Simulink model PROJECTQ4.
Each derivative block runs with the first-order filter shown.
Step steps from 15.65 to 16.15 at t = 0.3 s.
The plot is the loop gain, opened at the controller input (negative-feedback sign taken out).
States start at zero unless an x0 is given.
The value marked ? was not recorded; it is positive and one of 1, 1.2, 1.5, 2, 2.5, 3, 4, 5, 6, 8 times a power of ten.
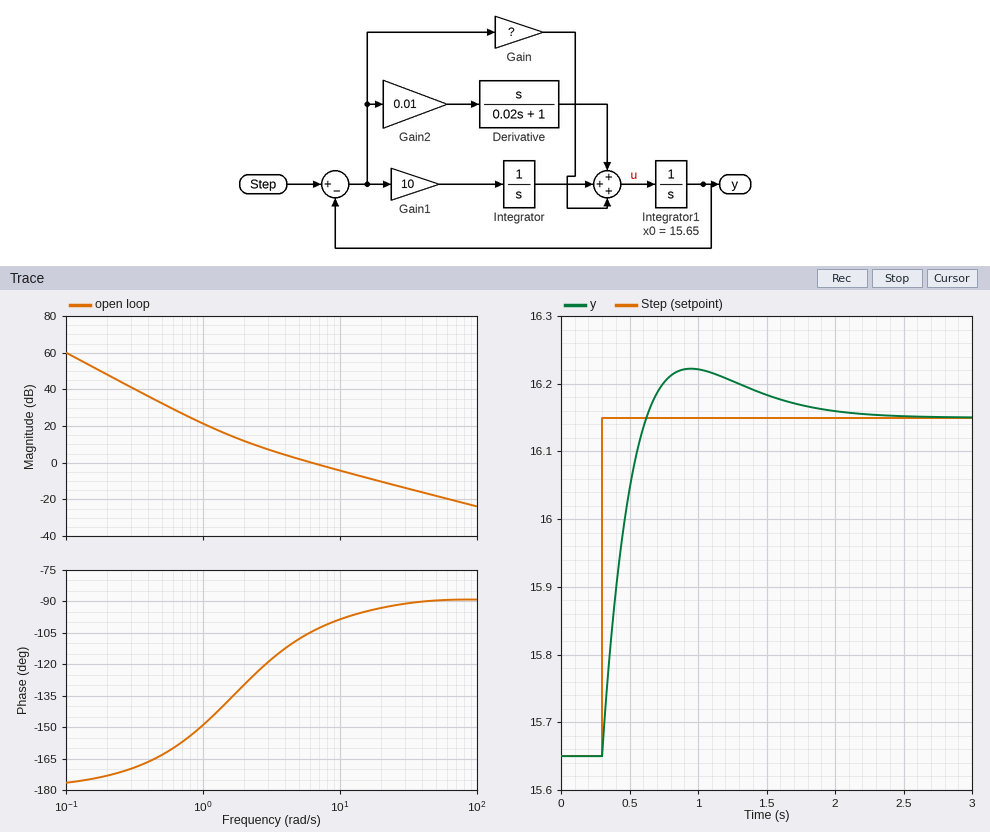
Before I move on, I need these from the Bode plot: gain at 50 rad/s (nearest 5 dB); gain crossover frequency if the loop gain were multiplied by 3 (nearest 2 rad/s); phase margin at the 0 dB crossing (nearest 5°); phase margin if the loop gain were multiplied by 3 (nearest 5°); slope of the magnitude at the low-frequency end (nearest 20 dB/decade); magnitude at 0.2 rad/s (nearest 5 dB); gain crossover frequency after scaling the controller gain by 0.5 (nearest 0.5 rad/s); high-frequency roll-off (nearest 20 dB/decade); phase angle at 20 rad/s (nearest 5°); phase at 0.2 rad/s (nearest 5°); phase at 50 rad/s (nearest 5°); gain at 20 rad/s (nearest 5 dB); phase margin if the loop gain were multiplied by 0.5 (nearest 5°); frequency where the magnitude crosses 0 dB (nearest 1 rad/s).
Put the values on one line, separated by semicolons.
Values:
-20 dB; 18 rad/s; 75°; 85°; -40 dB/decade; 50 dB; 3.5 rad/s; -20 dB/decade; -95°; -175°; -90°; -10 dB; 65°; 6 rad/s
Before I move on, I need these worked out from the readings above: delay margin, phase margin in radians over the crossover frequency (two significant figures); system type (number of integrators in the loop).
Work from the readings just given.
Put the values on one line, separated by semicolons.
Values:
0.22 s; 2
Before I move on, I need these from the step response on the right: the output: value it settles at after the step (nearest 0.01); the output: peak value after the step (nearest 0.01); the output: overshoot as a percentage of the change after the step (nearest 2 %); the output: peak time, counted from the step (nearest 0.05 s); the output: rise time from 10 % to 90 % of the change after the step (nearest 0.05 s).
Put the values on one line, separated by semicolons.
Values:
16.15; 16.22; 14 %; 0.65 s; 0.25 s
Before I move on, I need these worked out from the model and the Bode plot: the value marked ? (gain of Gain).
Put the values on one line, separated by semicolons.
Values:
6
